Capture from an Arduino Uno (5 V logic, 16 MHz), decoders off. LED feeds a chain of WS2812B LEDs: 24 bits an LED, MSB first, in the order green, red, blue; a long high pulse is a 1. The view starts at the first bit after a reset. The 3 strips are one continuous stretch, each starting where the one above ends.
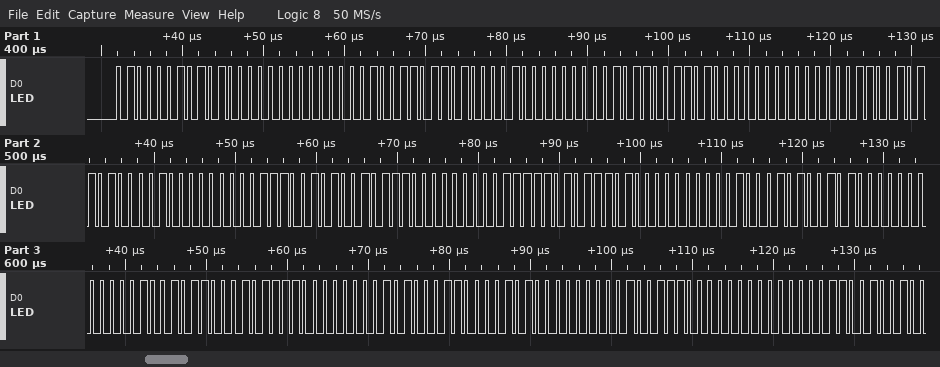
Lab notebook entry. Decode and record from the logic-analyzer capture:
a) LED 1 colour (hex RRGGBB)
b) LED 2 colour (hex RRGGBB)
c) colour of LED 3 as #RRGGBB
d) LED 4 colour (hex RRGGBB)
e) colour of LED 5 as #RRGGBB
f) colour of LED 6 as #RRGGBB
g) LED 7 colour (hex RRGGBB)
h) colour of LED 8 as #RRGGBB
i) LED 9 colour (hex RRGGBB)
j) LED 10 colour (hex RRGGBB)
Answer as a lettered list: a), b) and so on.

a) #A04200
b) #A14D00
c) #A05900
d) #A16500
e) #977200
f) #747D00
g) #508A00
h) #2F9600
i) #0AA300
j) #009C0C
